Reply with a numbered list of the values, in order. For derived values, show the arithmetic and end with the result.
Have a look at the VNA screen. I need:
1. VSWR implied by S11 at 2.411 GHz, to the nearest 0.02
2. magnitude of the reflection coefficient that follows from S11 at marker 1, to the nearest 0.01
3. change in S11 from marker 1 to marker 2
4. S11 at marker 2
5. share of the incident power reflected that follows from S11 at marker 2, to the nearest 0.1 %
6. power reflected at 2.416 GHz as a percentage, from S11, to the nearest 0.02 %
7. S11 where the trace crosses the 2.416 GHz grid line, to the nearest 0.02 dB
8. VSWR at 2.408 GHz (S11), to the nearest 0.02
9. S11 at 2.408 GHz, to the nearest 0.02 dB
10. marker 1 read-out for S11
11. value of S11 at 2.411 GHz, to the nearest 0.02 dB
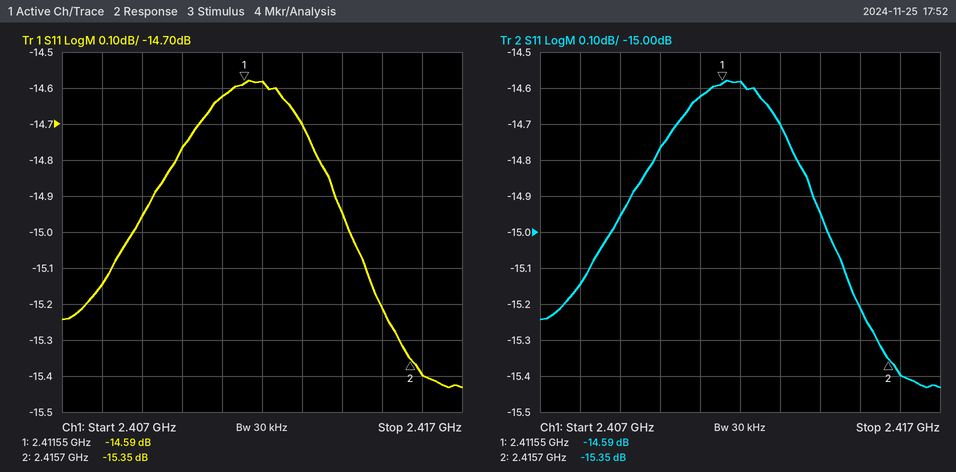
1. |Γ| = 10^(-14.62/20) = 0.1858; VSWR = (1 + 0.1858)/(1 − 0.1858) ≈ 1.46
2. 10^(-14.59/20) ≈ 0.19
3. -15.35 − (-14.59) = -0.76 dB
4. -15.35 dB
5. 10^(-15.35/10) ≈ 2.9 %
6. 10^(-15.4/10) ≈ 2.88 %
7. -15.40 dB
8. |Γ| = 10^(-15.14/20) = 0.1750; VSWR = (1 + 0.1750)/(1 − 0.1750) ≈ 1.42
9. -15.14 dB
10. -14.59 dB
11. -14.62 dB
